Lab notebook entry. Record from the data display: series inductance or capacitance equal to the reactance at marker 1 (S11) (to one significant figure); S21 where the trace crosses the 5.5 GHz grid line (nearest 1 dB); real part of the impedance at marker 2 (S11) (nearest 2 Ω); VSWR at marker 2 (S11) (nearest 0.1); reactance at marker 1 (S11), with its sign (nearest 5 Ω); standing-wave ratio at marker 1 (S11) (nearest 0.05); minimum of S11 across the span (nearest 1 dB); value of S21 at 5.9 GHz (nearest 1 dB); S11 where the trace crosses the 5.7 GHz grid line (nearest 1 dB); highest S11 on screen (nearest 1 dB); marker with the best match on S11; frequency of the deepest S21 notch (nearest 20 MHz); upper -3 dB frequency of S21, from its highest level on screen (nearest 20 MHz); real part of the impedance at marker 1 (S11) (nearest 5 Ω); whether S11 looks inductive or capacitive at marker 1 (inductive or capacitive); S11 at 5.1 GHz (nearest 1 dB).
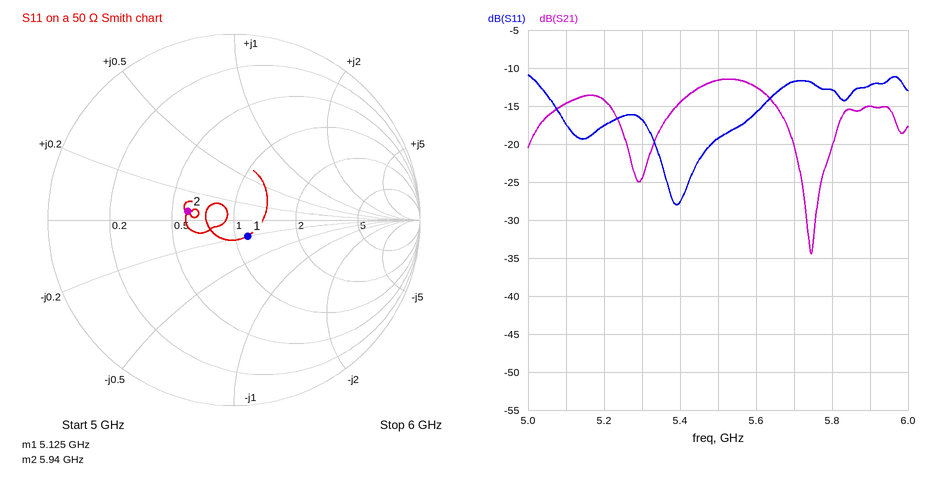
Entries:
3 pF
-12 dB
30 Ω
1.7
-10 Ω
1.25
-28 dB
-15 dB
-12 dB
-11 dB
marker 1
5.74 GHz
5.64 GHz
55 Ω
capacitive
-17 dB
